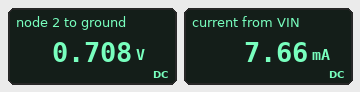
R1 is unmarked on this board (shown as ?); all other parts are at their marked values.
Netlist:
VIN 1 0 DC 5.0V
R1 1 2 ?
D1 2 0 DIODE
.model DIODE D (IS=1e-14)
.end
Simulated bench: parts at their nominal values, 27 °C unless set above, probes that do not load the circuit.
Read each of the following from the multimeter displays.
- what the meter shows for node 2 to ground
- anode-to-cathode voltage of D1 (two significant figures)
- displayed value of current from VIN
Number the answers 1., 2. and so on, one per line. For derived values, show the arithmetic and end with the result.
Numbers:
1. 0.708 V
2. 708 mV = 710 mV
3. 7.66 mA
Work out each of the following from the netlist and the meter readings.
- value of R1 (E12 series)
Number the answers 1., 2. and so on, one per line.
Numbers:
1. 560 Ω
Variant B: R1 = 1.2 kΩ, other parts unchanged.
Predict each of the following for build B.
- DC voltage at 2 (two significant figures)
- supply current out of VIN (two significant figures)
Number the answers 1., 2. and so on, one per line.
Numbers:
1. 690 mV
2. 3.6 mA
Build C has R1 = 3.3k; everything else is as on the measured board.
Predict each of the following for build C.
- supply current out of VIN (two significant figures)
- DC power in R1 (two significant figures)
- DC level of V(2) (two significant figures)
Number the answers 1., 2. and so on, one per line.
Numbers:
1. 1.3 mA
2. 5.7 mW
3. 660 mV
